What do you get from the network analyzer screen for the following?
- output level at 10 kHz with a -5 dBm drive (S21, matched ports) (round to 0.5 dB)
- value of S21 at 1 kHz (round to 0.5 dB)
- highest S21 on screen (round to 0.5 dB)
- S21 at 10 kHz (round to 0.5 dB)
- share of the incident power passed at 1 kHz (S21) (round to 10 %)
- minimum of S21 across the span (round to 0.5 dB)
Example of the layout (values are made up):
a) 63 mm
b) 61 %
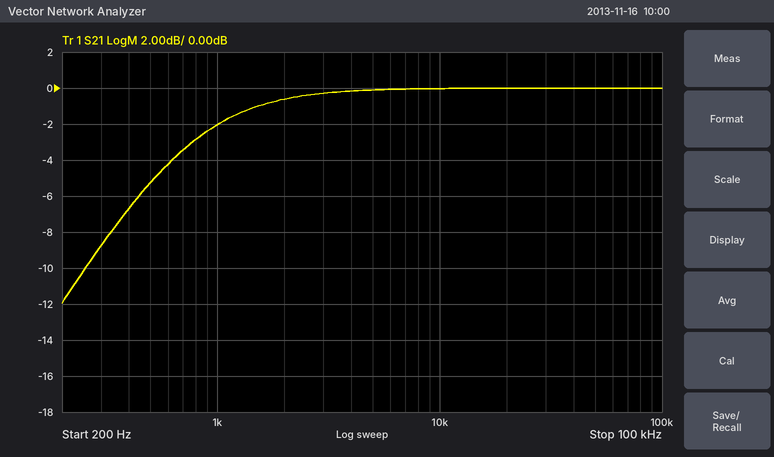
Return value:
a) -5.0 dBm
b) -2.0 dB
c) 0.0 dB
d) 0.0 dB
e) 60 %
f) -12.0 dB
